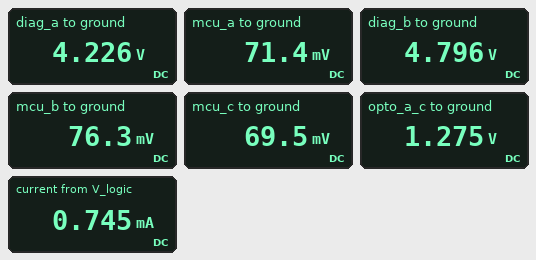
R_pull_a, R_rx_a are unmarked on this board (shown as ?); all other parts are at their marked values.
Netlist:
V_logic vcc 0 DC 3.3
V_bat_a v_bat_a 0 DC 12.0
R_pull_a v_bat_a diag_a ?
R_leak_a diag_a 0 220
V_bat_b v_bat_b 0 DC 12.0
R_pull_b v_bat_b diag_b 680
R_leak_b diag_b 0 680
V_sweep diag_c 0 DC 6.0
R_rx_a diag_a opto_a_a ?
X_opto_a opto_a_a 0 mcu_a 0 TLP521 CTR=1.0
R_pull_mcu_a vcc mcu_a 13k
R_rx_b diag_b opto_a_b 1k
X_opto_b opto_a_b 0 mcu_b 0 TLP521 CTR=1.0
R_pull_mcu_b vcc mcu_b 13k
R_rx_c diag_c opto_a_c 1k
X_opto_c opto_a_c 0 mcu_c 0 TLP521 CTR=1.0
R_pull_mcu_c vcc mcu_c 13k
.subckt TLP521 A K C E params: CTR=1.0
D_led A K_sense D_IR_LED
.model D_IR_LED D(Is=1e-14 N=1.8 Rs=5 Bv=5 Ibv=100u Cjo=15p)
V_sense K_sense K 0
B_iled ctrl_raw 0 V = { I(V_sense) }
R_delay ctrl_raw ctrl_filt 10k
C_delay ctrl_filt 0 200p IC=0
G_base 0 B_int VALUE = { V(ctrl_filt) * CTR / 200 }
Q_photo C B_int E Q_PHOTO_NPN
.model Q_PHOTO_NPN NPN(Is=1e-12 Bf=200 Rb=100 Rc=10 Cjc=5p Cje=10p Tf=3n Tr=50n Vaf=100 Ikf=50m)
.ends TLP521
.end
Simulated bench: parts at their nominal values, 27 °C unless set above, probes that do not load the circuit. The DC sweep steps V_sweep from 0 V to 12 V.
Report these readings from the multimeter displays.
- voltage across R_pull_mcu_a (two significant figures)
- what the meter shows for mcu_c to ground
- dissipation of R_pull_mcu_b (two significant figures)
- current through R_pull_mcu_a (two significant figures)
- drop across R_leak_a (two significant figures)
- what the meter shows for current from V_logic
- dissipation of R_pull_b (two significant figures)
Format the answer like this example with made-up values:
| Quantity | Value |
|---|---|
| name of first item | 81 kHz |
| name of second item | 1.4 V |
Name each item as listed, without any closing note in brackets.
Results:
| Quantity | Value |
|---|---|
| voltage across R_pull_mcu_a | 3.2 V |
| what the meter shows for mcu_c to ground | 69.5 mV |
| dissipation of R_pull_mcu_b | 800 µW |
| current through R_pull_mcu_a | 250 µA |
| drop across R_leak_a | 4.2 V |
| what the meter shows for current from V_logic | 0.745 mA |
| dissipation of R_pull_b | 76 mW |
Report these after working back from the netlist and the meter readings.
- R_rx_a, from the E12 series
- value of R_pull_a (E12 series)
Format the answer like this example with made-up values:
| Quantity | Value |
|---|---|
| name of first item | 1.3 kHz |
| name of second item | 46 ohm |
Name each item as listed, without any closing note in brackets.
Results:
| Quantity | Value |
|---|---|
| R_rx_a, from the E12 series | 680 Ω |
| value of R_pull_a | 330 Ω |
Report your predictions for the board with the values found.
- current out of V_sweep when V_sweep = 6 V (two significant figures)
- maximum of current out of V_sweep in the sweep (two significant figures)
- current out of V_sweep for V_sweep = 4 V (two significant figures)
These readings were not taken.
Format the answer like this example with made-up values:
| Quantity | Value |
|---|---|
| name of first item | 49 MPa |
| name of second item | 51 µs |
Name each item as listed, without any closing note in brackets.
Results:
| Quantity | Value |
|---|---|
| current out of V_sweep when V_sweep = 6 V | 4.7 mA |
| maximum of current out of V_sweep in the sweep | 11 mA |
| current out of V_sweep for V_sweep = 4 V | 2.8 mA |
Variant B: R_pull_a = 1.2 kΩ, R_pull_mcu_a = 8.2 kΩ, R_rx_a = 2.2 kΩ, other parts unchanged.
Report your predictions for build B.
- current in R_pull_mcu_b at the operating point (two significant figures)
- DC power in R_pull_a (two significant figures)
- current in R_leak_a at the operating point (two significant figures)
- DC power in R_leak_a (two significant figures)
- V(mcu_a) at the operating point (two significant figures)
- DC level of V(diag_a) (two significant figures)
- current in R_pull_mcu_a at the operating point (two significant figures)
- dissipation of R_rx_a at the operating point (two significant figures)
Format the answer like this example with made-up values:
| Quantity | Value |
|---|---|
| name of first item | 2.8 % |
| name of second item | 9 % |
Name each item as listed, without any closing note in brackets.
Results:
| Quantity | Value |
|---|---|
| current in R_pull_mcu_b at the operating point | 250 µA |
| DC power in R_pull_a | 87 mW |
| current in R_leak_a at the operating point | 8.2 mA |
| DC power in R_leak_a | 15 mW |
| V(mcu_a) at the operating point | 790 mV |
| DC level of V(diag_a) | 1.8 V |
| current in R_pull_mcu_a at the operating point | 310 µA |
| dissipation of R_rx_a at the operating point | 210 µW |
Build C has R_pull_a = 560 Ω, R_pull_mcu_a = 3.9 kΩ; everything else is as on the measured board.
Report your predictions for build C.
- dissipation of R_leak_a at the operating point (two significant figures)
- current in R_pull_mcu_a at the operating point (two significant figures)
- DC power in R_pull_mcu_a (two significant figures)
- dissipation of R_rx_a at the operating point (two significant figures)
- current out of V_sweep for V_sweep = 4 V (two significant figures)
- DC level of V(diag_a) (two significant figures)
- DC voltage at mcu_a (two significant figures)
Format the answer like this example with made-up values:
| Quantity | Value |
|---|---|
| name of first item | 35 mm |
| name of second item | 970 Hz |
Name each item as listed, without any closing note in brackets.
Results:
| Quantity | Value |
|---|---|
| dissipation of R_leak_a at the operating point | 40 mW |
| current in R_pull_mcu_a at the operating point | 810 µA |
| DC power in R_pull_mcu_a | 2.6 mW |
| dissipation of R_rx_a at the operating point | 4.5 mW |
| current out of V_sweep for V_sweep = 4 V | 2.8 mA |
| DC level of V(diag_a) | 3.0 V |
| DC voltage at mcu_a | 130 mV |
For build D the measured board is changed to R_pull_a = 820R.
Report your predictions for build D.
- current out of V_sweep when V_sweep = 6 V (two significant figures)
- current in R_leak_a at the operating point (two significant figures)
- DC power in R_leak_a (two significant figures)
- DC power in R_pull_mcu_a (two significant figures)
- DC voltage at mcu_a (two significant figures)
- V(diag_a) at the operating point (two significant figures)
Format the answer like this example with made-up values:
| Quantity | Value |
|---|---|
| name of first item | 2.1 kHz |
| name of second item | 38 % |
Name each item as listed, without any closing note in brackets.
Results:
| Quantity | Value |
|---|---|
| current out of V_sweep when V_sweep = 6 V | 4.7 mA |
| current in R_leak_a at the operating point | 10 mA |
| DC power in R_leak_a | 23 mW |
| DC power in R_pull_mcu_a | 790 µW |
| DC voltage at mcu_a | 98 mV |
| V(diag_a) at the operating point | 2.3 V |
